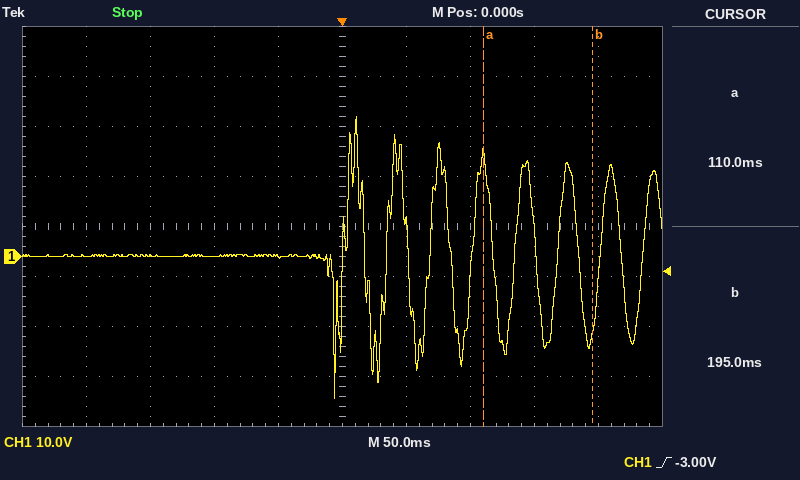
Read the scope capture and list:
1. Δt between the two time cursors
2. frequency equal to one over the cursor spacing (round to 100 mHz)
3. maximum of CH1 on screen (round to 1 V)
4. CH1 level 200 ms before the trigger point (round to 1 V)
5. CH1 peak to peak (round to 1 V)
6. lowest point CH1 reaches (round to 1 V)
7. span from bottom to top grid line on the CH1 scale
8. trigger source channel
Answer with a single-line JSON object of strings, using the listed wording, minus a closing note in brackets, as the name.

{"Δt between the two time cursors": "85 ms", "frequency equal to one over the cursor spacing": "11.8 Hz", "maximum of CH1 on screen": "28 V", "CH1 level 200 ms before the trigger point": "0 V", "CH1 peak to peak": "56 V", "lowest point CH1 reaches": "-28 V", "span from bottom to top grid line on the CH1 scale": "80 V", "trigger source channel": "CH1"}
